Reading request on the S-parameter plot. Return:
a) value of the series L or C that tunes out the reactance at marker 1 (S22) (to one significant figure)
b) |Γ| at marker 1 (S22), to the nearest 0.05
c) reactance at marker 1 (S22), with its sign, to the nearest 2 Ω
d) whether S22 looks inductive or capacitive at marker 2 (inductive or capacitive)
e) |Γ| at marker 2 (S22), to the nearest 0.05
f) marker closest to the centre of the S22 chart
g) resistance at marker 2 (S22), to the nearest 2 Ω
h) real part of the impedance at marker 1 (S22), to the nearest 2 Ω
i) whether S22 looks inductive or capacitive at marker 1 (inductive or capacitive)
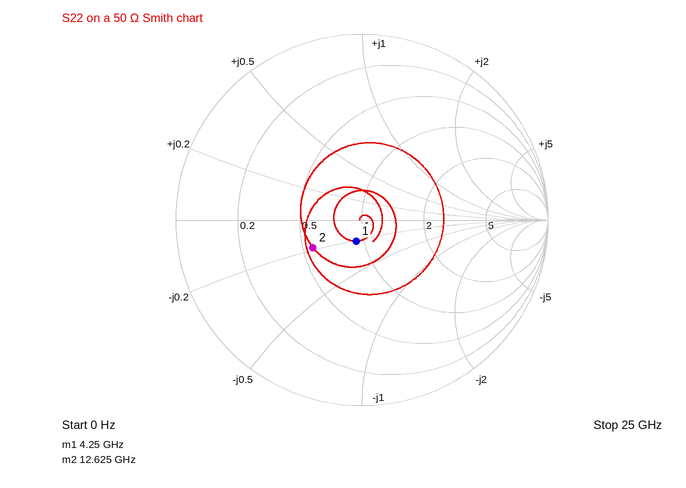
400 pH
0.10
-10 Ω
capacitive
0.30
marker 1
28 Ω
46 Ω
capacitive
